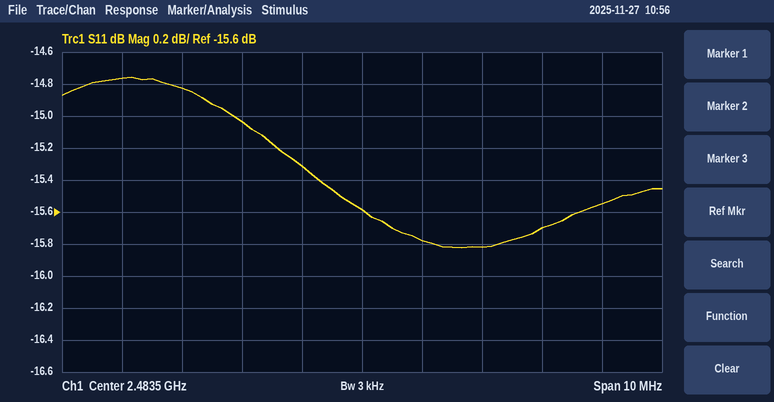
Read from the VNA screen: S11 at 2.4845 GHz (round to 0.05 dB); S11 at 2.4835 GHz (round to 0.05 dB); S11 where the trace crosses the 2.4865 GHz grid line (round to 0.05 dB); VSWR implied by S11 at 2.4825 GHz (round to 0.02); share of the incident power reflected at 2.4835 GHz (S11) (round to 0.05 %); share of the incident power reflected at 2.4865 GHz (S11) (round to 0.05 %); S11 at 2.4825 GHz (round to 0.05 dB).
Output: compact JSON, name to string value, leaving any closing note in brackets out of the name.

{"S11 at 2.4845 GHz": "-15.80 dB", "S11 at 2.4835 GHz": "-15.60 dB", "S11 where the trace crosses the 2.4865 GHz grid line": "-15.70 dB", "VSWR implied by S11 at 2.4825 GHz": "1.42", "share of the incident power reflected at 2.4835 GHz (S11)": "2.75 %", "share of the incident power reflected at 2.4865 GHz (S11)": "2.70 %", "S11 at 2.4825 GHz": "-15.30 dB"}
